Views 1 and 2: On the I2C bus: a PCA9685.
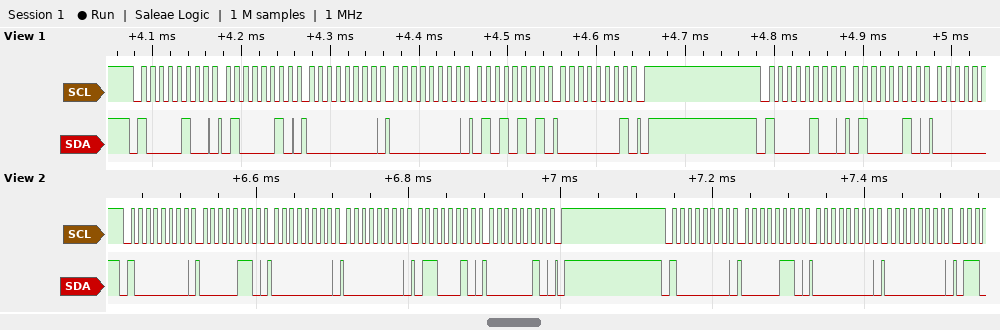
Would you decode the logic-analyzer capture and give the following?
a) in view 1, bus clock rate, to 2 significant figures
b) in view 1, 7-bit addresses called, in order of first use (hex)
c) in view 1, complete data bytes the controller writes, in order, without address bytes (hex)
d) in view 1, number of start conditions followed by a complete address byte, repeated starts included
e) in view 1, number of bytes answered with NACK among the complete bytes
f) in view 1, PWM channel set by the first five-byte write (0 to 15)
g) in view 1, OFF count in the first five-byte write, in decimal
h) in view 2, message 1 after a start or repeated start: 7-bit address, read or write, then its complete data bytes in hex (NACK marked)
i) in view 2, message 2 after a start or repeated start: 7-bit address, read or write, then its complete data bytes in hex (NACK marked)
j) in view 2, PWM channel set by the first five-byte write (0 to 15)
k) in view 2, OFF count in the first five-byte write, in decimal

100 kHz
0x42
42 00 00 55 01 42
2
0
15
341
0x40 write: 06 00 00 62 02
0x40 write: 06 00 00
0
610
